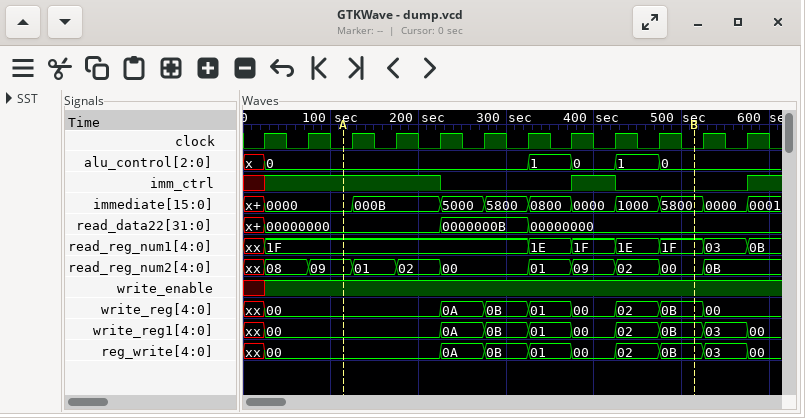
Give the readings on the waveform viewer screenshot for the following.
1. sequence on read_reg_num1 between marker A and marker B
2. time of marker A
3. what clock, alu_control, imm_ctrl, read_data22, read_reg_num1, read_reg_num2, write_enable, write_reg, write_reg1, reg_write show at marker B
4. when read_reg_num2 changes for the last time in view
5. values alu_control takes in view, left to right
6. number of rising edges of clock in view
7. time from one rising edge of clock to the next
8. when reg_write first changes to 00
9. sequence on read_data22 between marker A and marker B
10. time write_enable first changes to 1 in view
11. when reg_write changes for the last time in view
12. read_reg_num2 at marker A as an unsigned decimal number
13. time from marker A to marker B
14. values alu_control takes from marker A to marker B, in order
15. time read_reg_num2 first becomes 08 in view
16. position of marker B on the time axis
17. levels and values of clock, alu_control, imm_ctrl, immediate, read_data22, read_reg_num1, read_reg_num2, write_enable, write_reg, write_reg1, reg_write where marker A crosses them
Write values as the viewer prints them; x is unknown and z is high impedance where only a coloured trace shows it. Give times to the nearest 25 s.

1F, 1E, 1F, 1E, 1F
125 s
clock=0, alu_control=0, imm_ctrl=0, read_data22=00000000, read_reg_num1=1F, read_reg_num2=00, write_enable=1, write_reg=0B, write_reg1=0B, reg_write=0B
525 s
x, 0, 1, 0, 1, 0
12
50 s
25 s
00000000, 0000000B, 00000000
25 s
575 s
9
400 s
0, 1, 0, 1, 0
25 s
525 s
clock=0, alu_control=0, imm_ctrl=1, immediate=0000, read_data22=00000000, read_reg_num1=1F, read_reg_num2=09, write_enable=1, write_reg=00, write_reg1=00, reg_write=00
